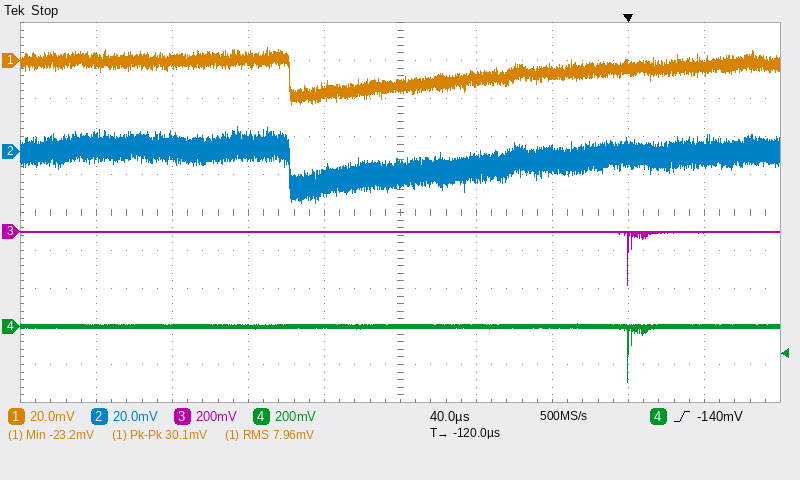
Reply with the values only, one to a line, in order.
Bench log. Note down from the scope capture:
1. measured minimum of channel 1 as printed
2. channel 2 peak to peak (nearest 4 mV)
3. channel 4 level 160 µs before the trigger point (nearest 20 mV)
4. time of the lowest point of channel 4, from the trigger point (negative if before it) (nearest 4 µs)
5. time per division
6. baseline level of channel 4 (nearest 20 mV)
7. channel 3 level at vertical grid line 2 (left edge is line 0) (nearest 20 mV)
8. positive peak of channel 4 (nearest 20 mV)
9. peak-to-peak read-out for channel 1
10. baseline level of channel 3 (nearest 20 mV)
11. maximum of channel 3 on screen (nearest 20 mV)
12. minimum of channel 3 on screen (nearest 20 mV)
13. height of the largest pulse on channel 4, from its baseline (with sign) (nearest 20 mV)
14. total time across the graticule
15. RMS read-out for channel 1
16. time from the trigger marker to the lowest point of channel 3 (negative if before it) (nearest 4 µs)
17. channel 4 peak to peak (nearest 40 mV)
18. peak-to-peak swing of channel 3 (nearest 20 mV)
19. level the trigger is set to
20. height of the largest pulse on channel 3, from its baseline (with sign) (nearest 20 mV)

-23.2 mV
40 mV
0 mV
0 µs
40 µs
0 mV
0 mV
20 mV
30.1 mV
0 mV
0 mV
-280 mV
-300 mV
400 µs
7.96 mV
0 µs
320 mV
280 mV
-140 mV
-280 mV
